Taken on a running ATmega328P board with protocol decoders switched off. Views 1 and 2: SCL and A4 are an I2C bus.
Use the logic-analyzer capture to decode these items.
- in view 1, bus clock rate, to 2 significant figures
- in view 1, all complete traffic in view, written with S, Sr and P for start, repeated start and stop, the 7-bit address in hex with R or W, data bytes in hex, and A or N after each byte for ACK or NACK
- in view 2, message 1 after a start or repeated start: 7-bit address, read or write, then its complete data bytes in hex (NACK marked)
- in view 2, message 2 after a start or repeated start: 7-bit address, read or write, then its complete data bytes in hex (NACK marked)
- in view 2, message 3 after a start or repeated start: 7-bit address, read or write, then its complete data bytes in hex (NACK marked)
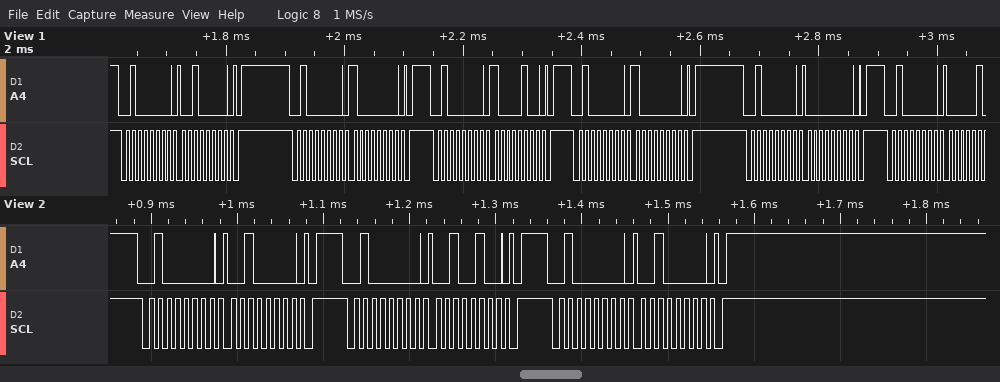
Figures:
100 kHz
S 20W A 20 A P S 20W A 80 A P S 20W A 84 A P S 20W A 80 A P S 20W A 00 A P S 20W A
0x20 write: 20
0x20 write: 24
0x20 write: 20
